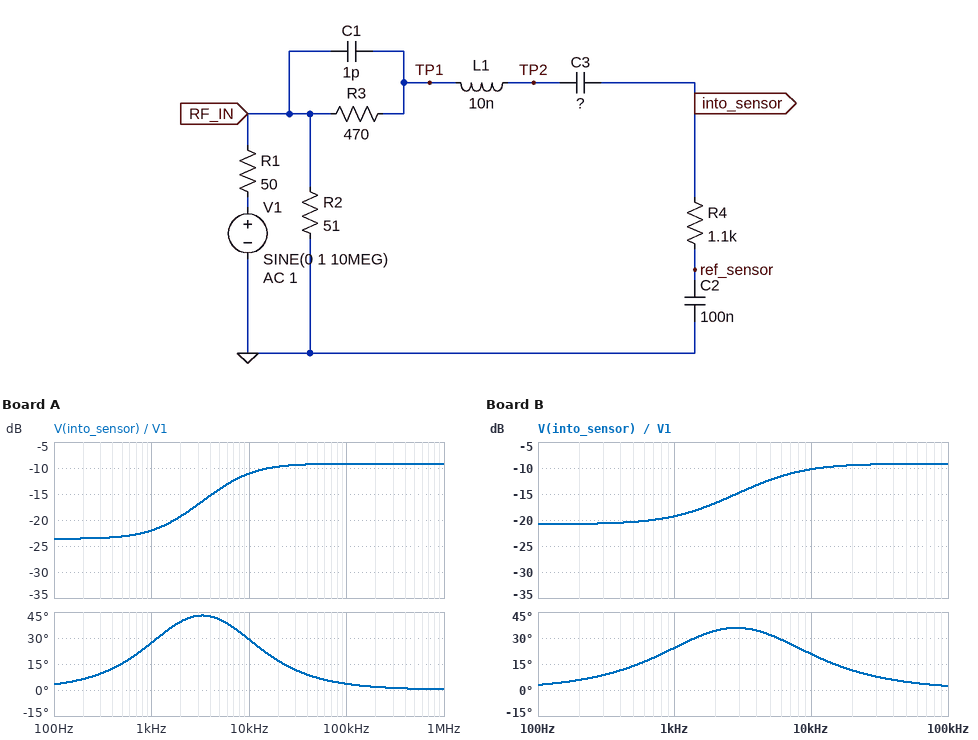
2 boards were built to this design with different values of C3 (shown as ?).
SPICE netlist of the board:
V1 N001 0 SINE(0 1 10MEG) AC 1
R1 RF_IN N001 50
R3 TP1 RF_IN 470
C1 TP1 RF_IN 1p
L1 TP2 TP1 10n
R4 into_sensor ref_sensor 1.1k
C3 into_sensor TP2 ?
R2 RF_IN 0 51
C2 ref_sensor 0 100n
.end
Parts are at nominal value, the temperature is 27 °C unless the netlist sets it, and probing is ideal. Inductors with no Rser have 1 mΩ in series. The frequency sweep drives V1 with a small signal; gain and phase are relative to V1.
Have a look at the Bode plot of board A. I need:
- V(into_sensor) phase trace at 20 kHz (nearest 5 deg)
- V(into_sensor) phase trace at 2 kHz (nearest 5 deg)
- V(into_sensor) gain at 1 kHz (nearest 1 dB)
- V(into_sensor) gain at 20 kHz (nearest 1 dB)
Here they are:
15 deg
40 deg
-22 dB
-10 dB
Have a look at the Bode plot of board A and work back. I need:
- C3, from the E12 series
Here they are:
15 nF
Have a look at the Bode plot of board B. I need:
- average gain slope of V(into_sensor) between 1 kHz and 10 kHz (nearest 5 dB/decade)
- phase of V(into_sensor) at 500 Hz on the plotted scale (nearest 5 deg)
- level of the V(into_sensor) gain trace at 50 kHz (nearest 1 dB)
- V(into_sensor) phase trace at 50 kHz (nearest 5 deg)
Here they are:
10 dB/decade
15 deg
-9 dB
5 deg
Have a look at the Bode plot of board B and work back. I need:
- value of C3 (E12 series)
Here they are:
22 nF
